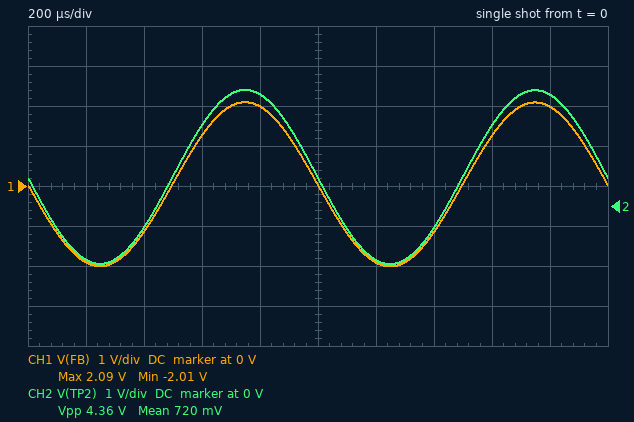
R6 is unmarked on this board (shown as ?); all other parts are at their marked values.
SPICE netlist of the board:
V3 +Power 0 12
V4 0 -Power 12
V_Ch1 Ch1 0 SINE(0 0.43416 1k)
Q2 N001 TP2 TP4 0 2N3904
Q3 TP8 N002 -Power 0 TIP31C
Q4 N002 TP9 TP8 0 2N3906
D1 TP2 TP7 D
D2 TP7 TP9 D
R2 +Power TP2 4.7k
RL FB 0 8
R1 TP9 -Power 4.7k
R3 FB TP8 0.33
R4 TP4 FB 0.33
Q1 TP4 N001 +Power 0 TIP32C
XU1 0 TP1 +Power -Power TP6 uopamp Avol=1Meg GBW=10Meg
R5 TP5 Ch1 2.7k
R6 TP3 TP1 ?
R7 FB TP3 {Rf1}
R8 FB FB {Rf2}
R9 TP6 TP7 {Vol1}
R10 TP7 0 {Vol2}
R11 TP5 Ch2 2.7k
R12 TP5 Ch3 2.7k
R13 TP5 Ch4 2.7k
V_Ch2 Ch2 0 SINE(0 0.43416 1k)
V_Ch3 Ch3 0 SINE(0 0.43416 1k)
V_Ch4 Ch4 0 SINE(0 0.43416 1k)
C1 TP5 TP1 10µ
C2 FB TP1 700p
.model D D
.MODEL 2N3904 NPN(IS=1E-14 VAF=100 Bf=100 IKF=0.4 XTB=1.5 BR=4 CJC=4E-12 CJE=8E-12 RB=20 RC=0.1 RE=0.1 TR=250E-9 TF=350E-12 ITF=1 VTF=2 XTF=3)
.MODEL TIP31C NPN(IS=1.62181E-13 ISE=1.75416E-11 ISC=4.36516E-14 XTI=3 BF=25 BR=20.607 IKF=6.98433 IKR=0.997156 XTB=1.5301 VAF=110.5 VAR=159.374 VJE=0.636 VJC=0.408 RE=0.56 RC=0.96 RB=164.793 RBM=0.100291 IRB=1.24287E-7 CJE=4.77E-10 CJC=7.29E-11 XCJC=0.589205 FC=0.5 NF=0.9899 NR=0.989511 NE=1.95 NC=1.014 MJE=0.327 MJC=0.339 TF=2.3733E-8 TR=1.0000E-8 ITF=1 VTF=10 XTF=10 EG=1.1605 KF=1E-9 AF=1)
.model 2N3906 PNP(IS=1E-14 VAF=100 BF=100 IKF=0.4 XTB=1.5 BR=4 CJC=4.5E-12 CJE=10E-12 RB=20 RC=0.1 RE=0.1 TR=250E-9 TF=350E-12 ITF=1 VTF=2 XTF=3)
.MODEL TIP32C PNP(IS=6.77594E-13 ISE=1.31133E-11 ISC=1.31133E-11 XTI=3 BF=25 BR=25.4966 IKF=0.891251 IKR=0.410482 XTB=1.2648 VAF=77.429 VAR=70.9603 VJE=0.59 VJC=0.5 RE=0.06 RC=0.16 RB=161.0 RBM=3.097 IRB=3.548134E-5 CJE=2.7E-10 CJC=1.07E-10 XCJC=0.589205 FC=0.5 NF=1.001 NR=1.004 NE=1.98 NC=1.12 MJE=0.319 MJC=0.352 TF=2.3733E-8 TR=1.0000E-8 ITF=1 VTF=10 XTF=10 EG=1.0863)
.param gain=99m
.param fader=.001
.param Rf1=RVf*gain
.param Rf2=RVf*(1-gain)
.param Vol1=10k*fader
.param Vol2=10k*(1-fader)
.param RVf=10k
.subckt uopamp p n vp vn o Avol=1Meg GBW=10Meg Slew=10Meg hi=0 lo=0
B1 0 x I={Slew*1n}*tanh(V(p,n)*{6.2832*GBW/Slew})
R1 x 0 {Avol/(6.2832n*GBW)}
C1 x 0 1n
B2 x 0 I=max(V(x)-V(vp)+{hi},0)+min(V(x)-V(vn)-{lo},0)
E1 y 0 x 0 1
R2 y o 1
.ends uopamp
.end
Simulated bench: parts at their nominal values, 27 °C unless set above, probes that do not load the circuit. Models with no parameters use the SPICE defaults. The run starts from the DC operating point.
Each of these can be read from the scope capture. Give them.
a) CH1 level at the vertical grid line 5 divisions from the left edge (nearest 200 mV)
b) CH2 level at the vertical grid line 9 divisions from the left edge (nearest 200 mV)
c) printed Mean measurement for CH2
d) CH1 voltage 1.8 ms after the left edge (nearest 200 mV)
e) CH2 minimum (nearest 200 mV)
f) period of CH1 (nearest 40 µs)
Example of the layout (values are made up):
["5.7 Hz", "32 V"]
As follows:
["0 V", "2.8 V", "720 mV", "2.0 V", "-1.4 V", "1.00 ms"]
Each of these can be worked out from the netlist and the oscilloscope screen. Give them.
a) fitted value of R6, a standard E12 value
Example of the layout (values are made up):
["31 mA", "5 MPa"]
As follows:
["2.2 kΩ"]
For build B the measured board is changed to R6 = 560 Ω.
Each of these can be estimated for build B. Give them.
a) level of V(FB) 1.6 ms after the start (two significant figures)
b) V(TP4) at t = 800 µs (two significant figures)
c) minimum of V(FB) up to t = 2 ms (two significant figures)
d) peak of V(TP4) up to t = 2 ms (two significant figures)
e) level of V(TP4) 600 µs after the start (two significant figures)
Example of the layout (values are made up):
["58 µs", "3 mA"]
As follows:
["620 mV", "1.0 V", "-980 mV", "1.1 V", "650 mV"]
